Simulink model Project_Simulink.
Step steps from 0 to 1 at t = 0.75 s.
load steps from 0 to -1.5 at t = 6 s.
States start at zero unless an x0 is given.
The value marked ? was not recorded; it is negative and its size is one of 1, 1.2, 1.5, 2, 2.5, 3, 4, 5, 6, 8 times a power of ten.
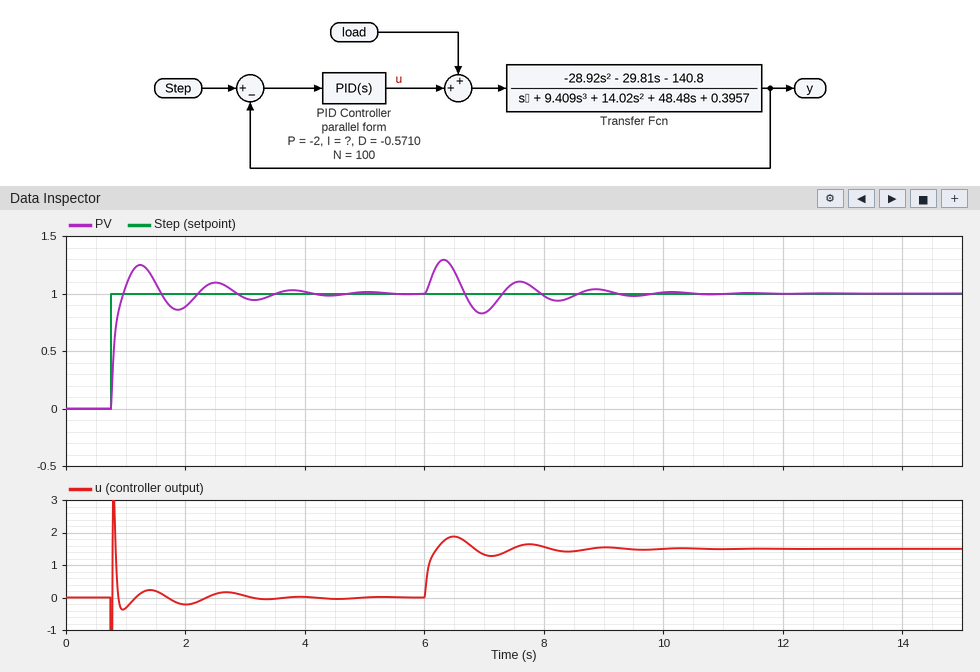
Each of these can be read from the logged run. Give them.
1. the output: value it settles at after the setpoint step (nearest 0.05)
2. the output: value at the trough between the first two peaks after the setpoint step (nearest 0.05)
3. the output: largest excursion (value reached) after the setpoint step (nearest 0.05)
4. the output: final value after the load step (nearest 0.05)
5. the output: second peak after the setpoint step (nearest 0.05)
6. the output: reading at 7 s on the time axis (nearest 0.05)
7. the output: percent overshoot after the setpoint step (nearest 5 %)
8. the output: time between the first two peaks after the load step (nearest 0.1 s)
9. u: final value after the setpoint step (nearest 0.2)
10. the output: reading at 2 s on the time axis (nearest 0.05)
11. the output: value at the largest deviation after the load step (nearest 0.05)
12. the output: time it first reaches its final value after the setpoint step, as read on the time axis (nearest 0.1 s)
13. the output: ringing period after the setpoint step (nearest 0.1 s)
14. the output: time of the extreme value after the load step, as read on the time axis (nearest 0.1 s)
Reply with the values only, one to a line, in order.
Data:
1.00
0.85
1.25
1.00
1.10
0.85
25 %
1.3 s
0.0
0.90
1.30
1.0 s
1.3 s
6.3 s
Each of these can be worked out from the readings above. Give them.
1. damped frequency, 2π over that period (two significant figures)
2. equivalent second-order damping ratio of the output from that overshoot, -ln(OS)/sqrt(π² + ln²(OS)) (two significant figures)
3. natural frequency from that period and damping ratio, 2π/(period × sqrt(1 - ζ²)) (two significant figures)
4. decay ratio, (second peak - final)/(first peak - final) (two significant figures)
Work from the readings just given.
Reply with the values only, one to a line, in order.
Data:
4.8 rad/s
0.40
5.3 rad/s
0.40
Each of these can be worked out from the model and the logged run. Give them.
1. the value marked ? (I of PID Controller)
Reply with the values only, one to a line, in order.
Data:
-20
